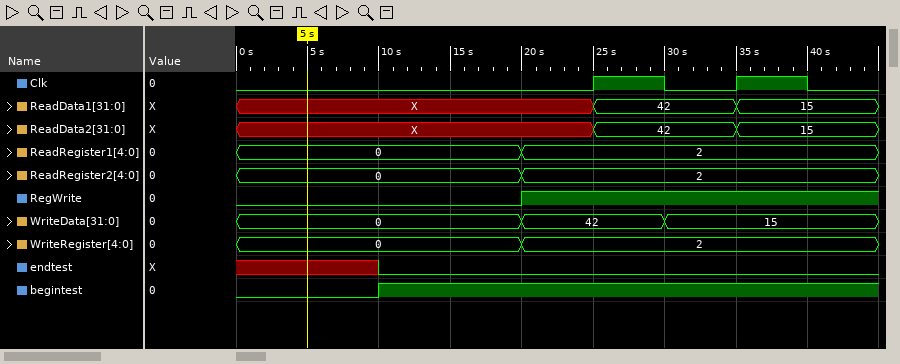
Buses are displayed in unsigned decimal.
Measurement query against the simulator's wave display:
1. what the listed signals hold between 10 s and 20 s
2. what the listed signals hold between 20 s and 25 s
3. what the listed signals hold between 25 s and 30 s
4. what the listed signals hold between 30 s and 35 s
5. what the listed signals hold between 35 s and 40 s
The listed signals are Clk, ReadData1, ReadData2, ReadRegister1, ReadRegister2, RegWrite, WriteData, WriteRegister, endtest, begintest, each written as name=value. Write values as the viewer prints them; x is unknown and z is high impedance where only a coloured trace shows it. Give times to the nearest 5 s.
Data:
Clk=0, ReadData1=X, ReadData2=X, ReadRegister1=0, ReadRegister2=0, RegWrite=0, WriteData=0, WriteRegister=0, endtest=0, begintest=1
Clk=0, ReadData1=X, ReadData2=X, ReadRegister1=2, ReadRegister2=2, RegWrite=1, WriteData=42, WriteRegister=2, endtest=0, begintest=1
Clk=1, ReadData1=42, ReadData2=42, ReadRegister1=2, ReadRegister2=2, RegWrite=1, WriteData=42, WriteRegister=2, endtest=0, begintest=1
Clk=0, ReadData1=42, ReadData2=42, ReadRegister1=2, ReadRegister2=2, RegWrite=1, WriteData=15, WriteRegister=2, endtest=0, begintest=1
Clk=1, ReadData1=15, ReadData2=15, ReadRegister1=2, ReadRegister2=2, RegWrite=1, WriteData=15, WriteRegister=2, endtest=0, begintest=1
